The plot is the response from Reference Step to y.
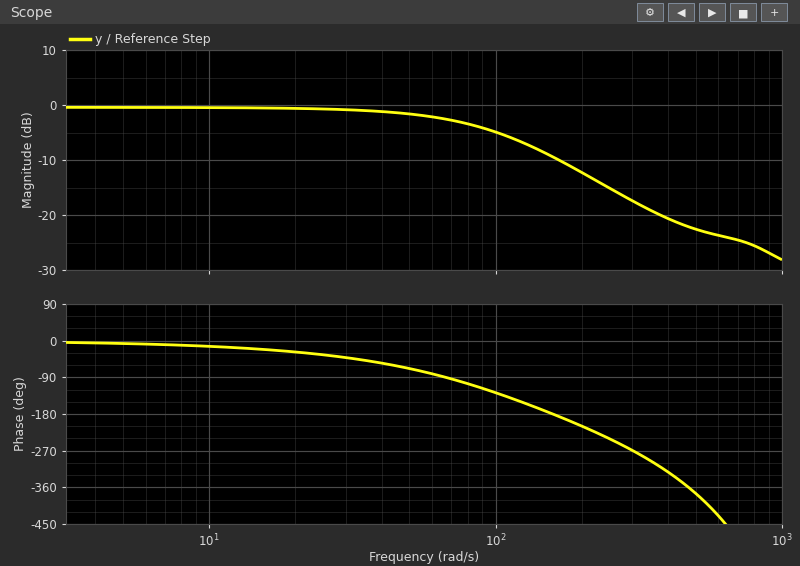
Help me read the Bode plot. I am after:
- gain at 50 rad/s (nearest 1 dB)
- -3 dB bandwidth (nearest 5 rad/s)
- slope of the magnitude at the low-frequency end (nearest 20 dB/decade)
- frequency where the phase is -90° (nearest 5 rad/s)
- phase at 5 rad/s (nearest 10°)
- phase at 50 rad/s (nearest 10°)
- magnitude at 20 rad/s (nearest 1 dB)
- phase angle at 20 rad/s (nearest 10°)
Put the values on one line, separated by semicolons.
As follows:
-2 dB; 80 rad/s; 0 dB/decade; 65 rad/s; -10°; -70°; -1 dB; -30°
